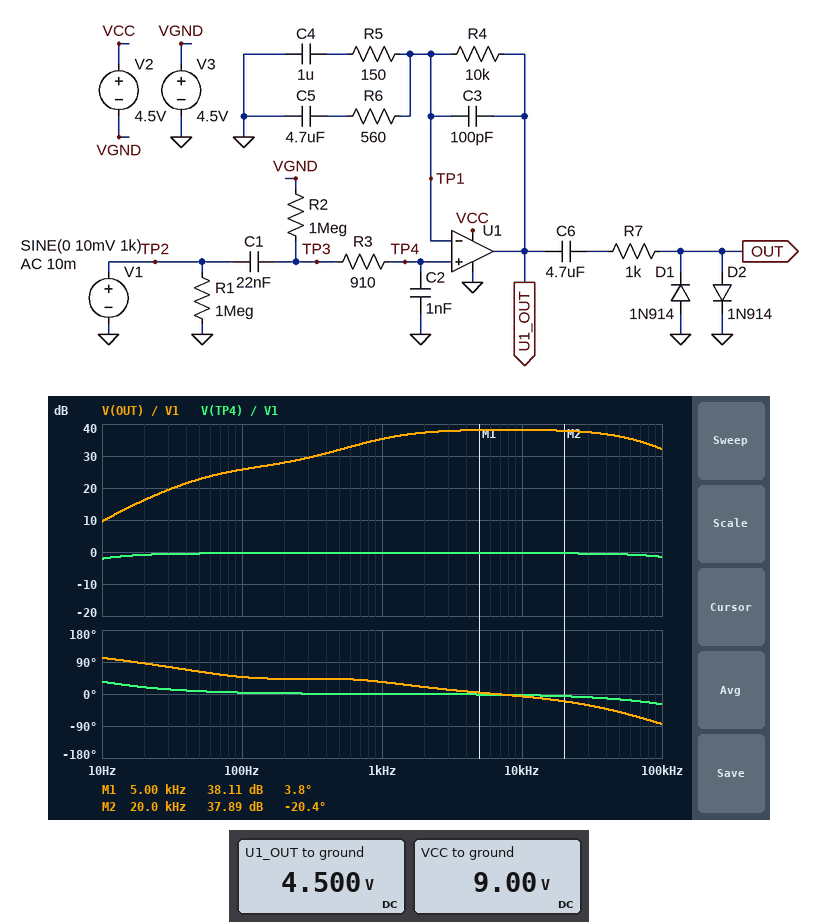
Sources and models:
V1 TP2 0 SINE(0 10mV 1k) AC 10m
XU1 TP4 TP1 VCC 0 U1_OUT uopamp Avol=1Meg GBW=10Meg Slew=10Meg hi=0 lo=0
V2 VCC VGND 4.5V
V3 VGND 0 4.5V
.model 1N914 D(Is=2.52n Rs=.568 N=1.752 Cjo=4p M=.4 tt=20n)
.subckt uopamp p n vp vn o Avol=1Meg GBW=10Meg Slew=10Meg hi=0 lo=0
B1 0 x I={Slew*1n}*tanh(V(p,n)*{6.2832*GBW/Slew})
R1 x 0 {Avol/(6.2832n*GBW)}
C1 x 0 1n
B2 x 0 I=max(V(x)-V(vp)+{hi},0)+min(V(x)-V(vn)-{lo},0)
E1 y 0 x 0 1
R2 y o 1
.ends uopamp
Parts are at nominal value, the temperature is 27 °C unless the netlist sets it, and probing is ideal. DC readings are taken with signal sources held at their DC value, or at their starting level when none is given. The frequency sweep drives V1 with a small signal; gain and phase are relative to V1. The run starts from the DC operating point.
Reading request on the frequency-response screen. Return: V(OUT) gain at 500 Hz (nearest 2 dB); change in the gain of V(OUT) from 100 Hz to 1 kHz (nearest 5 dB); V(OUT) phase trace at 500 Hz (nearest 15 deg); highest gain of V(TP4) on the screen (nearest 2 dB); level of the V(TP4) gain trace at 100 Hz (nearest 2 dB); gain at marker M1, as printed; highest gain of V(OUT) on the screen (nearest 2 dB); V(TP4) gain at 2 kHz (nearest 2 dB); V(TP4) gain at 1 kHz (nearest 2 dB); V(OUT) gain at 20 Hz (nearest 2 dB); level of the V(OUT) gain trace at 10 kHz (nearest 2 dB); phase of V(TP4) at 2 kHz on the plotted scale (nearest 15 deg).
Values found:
32 dB
10 dB
45 deg
0 dB
0 dB
38.11 dB
38 dB
0 dB
0 dB
16 dB
38 dB
0 deg
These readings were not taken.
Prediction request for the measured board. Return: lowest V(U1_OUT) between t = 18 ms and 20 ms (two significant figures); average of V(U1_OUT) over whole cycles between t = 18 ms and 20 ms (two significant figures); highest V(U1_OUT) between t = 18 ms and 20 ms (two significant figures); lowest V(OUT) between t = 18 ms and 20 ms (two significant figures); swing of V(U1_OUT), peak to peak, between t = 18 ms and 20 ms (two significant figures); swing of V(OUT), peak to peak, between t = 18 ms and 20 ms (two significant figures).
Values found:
3.9 V
4.5 V
5.1 V
-480 mV
1.2 V
960 mV
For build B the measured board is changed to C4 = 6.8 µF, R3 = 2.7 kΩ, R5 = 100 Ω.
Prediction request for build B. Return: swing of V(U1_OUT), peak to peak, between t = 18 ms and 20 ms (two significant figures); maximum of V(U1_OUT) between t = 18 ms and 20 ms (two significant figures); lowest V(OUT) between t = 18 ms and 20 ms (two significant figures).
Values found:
2.2 V
5.6 V
-560 mV
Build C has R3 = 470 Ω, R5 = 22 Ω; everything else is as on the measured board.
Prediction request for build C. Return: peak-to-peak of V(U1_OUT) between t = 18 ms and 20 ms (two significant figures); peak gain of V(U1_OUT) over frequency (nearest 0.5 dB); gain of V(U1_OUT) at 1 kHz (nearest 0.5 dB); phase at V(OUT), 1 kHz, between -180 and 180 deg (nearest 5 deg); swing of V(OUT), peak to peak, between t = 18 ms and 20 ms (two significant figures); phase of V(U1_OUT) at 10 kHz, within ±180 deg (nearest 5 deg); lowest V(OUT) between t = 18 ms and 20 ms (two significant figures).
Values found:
1.3 V
52.5 dB
36.5 dB
65 deg
1.0 V
5 deg
-500 mV
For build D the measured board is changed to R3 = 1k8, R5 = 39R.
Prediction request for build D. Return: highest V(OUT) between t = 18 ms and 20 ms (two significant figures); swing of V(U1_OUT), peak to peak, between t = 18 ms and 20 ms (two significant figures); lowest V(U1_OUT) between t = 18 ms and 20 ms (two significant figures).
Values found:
500 mV
1.3 V
3.8 V
